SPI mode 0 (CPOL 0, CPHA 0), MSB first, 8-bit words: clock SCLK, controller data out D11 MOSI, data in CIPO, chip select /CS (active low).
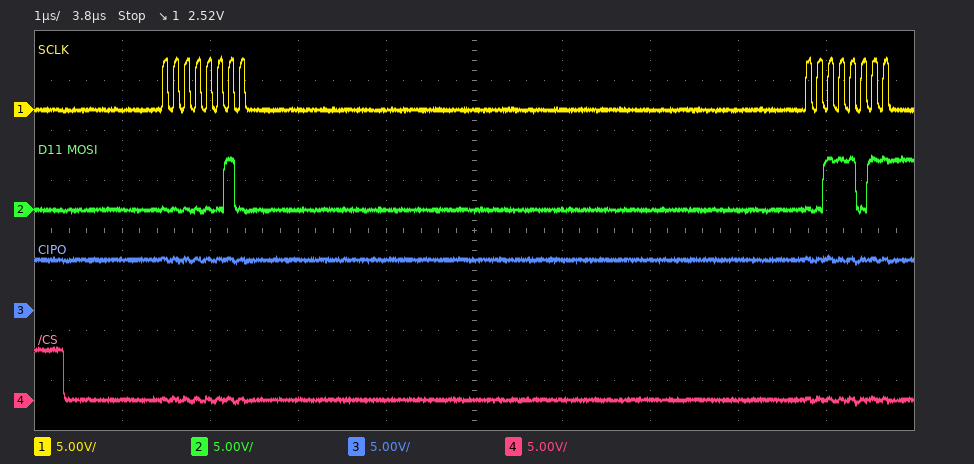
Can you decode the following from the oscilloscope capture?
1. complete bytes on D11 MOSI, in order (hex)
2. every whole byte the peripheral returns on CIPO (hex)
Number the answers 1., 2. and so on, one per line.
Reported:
1. 0x02 0x3B
2. 0xFF 0xFF
